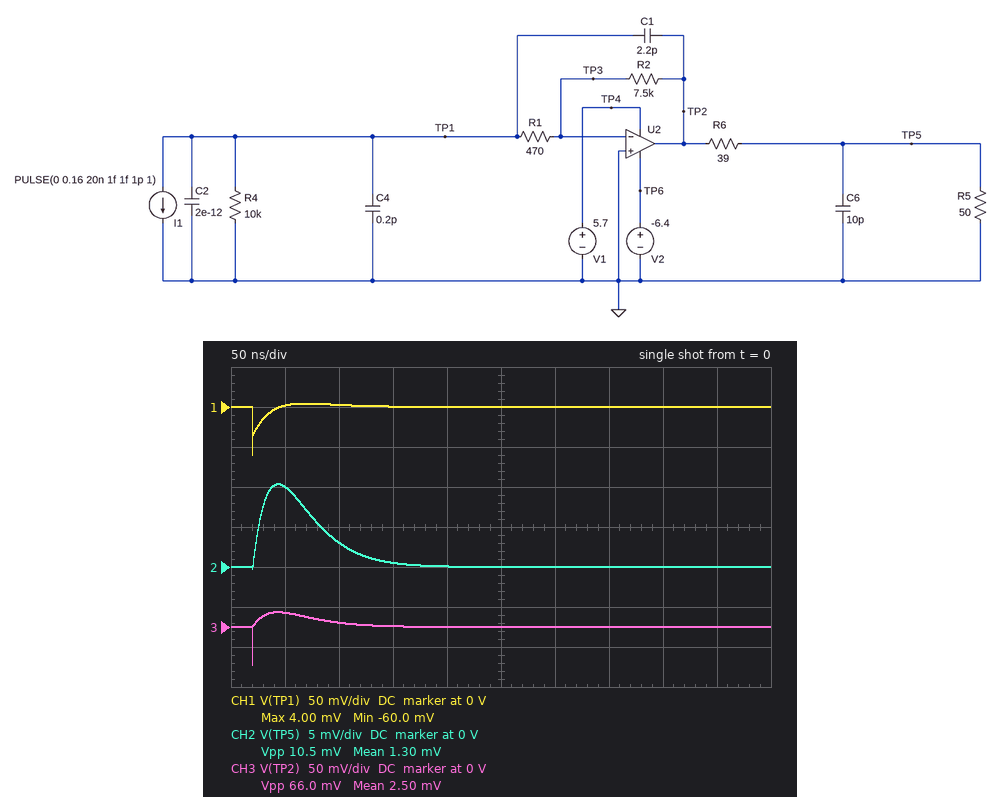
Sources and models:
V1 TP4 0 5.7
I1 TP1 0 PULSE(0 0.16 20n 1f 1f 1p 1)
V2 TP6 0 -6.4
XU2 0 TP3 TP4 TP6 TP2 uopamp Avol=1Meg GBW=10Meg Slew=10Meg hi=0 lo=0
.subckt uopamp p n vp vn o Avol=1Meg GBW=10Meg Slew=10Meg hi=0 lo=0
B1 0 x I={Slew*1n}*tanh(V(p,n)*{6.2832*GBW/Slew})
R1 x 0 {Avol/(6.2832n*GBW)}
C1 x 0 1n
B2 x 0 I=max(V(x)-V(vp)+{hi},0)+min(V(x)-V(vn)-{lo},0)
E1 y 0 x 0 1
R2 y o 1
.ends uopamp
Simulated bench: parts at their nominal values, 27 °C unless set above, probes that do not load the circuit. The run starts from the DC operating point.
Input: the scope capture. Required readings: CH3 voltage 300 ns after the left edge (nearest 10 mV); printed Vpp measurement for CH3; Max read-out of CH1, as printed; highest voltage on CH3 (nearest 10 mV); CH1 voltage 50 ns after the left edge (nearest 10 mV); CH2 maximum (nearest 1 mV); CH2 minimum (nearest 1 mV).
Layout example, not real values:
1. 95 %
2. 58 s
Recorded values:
1. 0 V
2. 66.0 mV
3. 4.00 mV
4. 20 mV
5. 0 V
6. 10 mV
7. 0 V
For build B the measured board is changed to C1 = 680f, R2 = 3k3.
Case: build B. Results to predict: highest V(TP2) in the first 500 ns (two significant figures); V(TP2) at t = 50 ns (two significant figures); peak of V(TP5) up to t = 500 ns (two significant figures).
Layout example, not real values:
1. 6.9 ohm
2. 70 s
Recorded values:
1. 15 mV
2. 9.1 mV
3. 8.3 mV
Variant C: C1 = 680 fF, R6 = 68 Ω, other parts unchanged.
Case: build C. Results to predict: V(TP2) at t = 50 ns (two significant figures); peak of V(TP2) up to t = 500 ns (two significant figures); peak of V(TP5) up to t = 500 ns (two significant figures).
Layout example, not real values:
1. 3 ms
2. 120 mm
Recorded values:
1. 21 mV
2. 24 mV
3. 10 mV
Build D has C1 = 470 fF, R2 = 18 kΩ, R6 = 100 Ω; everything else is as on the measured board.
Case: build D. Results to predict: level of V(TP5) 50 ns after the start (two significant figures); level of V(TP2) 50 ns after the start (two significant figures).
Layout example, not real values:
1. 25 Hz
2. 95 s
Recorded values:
1. 12 mV
2. 37 mV
